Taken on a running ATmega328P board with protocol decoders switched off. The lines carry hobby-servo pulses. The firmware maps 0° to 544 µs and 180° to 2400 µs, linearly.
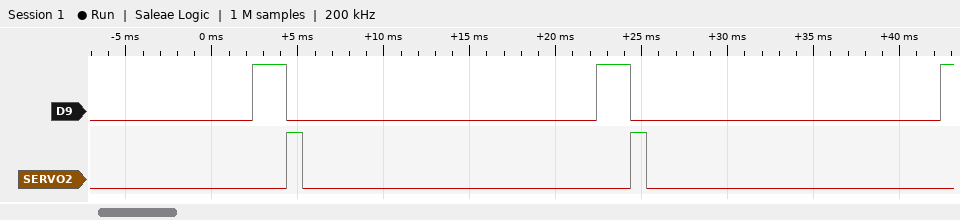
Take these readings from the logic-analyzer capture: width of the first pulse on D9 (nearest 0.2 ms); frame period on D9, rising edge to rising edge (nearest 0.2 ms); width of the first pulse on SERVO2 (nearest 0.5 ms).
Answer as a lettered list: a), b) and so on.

a) 2.0 ms
b) 20.0 ms
c) 1.0 ms
